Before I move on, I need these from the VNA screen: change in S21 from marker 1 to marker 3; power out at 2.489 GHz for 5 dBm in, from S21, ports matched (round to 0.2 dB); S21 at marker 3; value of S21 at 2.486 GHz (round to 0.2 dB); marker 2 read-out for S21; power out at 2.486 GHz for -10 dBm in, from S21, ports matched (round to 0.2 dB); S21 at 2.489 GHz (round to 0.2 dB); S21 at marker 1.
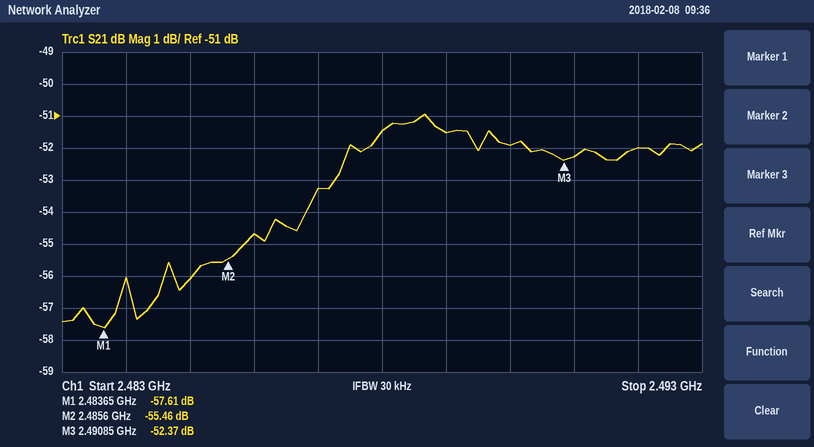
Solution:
5.24 dB
-46.6 dBm
-52.37 dB
-54.6 dB
-55.46 dB
-64.6 dBm
-51.6 dB
-57.61 dB
